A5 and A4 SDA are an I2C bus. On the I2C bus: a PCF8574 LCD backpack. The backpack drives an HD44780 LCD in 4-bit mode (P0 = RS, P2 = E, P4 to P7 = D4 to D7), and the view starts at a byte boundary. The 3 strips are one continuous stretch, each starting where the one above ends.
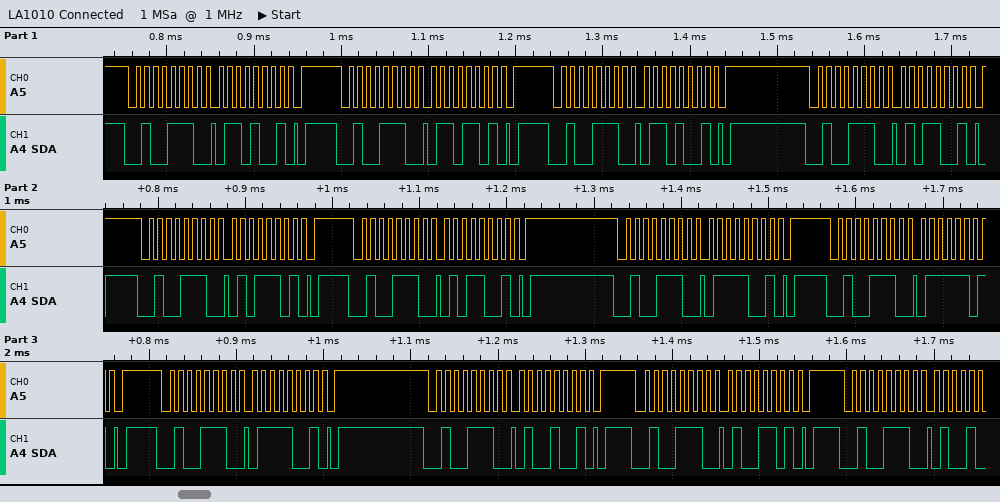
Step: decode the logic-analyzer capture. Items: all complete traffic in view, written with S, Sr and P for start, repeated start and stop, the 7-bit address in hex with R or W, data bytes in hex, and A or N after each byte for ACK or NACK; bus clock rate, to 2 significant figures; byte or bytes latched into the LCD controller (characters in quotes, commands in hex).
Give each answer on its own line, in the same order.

S 27W A 69 A P S 27W A 6D A P S 27W A 69 A P S 27W A 59 A P S 27W A 5D A P S 27W A 59 A P S 27W A 79 A P S 27W A 7D A P S 27W A 79 A P S 27W A 49 A P S 27W A 4D A P S 27W A
100 kHz
'e'
